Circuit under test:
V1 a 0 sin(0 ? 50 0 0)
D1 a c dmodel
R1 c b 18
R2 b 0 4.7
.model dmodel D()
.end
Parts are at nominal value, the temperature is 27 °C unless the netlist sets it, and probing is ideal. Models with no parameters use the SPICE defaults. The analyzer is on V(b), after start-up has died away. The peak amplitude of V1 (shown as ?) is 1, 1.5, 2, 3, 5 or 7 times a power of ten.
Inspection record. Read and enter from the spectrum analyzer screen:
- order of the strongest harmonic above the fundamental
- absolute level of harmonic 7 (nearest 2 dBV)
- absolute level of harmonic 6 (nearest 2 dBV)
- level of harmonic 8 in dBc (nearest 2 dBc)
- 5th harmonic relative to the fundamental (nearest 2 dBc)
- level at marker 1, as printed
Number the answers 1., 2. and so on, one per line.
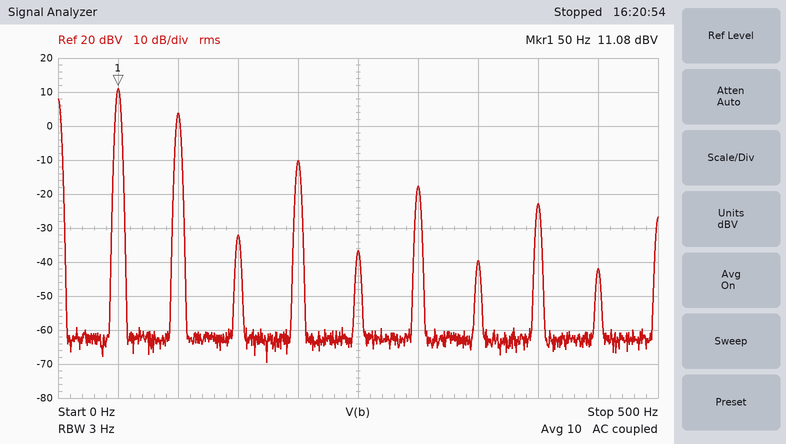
1. 2
2. -40 dBV
3. -18 dBV
4. -34 dBc
5. -48 dBc
6. 11.08 dBV
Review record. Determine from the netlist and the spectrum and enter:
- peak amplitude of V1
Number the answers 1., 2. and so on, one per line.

1. 50 V
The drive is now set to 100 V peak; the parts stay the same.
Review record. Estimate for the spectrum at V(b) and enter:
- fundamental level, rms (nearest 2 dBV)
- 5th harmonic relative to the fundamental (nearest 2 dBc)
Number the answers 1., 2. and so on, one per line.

1. 18 dBV
2. -54 dBc
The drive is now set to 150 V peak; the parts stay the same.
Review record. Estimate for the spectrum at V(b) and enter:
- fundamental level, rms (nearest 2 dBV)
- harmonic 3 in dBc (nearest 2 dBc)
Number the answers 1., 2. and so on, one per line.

1. 20 dBV
2. -52 dBc
